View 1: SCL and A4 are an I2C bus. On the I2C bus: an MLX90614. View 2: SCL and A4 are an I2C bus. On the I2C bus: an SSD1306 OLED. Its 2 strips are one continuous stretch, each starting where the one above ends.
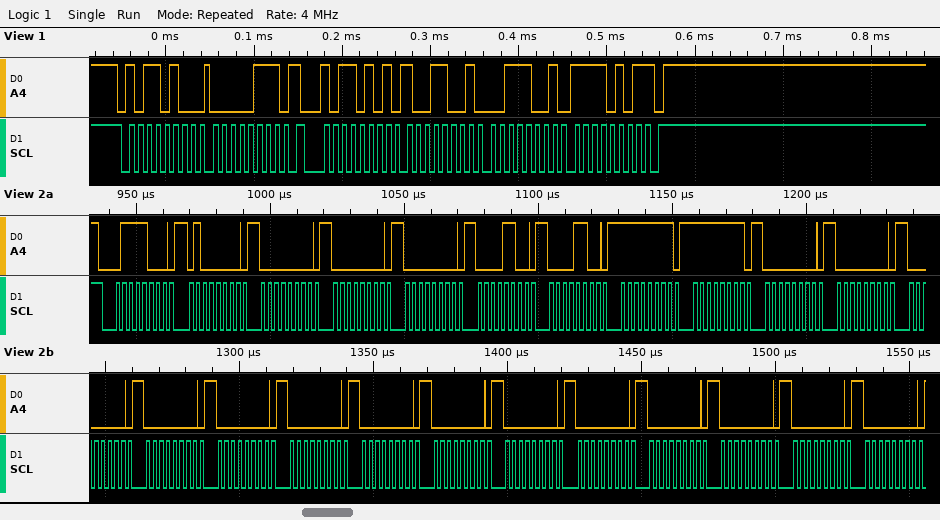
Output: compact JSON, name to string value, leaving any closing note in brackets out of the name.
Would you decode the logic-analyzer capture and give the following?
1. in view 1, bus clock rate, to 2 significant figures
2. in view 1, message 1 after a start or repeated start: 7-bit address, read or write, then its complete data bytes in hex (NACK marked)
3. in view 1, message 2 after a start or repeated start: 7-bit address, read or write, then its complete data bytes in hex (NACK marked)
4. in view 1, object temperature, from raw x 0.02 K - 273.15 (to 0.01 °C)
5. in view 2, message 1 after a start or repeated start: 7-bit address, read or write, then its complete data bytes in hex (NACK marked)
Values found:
{"in view 1, bus clock rate, to 2 significant figures": "100 kHz", "in view 1, message 1 after a start or repeated start: 7-bit address, read or write, then its complete data bytes in hex": "0x5A write: 07", "in view 1, message 2 after a start or repeated start: 7-bit address, read or write, then its complete data bytes in hex": "0x5A read: 99 39 F5 NACK", "in view 1, object temperature, from raw x 0.02 K - 273.15": "21.75 °C", "in view 2, message 1 after a start or repeated start: 7-bit address, read or write, then its complete data bytes in hex": "0x3C write: 40 00 00 00 0C 0C FF FF 00 00 00 00 00 00 00 00 00 00 00 00 00 00"}
